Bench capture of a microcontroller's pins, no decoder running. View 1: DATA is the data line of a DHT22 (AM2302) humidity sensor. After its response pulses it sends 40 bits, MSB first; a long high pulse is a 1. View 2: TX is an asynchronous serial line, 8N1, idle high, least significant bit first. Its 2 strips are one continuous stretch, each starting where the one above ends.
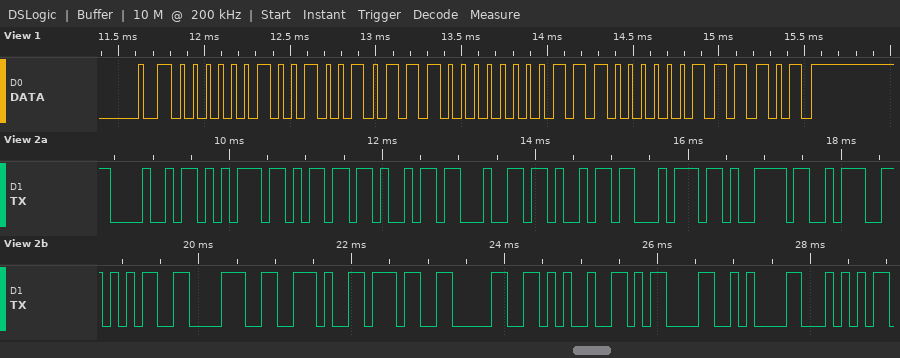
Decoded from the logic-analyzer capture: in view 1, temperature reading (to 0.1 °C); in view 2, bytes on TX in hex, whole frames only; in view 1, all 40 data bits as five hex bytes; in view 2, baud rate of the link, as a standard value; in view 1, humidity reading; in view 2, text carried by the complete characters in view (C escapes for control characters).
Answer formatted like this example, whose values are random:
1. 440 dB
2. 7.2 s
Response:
1. -11.2 °C
2. 48 75 6D 69 64 69 74 79 3A 35 38 2E 37 30 25 0D 0A 54
3. 02 4B 80 70 3D
4. 9600 baud
5. 58.7 %
6. "Humidity:58.70%\r\nT"
